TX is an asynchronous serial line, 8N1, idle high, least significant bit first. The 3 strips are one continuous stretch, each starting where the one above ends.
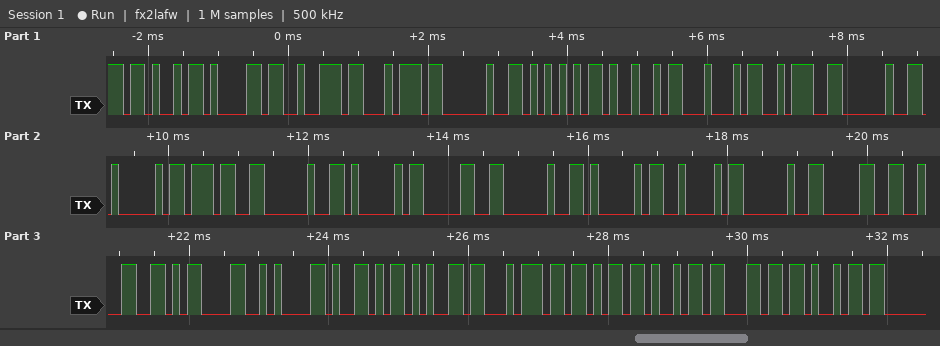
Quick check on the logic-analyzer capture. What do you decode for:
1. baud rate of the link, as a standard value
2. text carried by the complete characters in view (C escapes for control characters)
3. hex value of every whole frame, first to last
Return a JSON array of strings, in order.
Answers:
["9600 baud", "\"Kart UID: A7 A0 AB 02\\r\\nYetkili\"", "4B 61 72 74 20 55 49 44 3A 20 41 37 20 41 30 20 41 42 20 30 32 0D 0A 59 65 74 6B 69 6C 69"]
